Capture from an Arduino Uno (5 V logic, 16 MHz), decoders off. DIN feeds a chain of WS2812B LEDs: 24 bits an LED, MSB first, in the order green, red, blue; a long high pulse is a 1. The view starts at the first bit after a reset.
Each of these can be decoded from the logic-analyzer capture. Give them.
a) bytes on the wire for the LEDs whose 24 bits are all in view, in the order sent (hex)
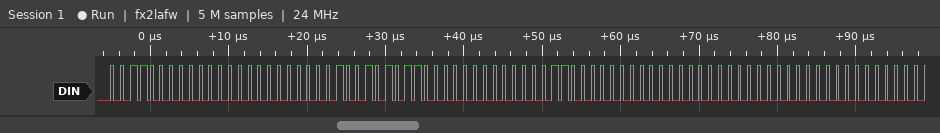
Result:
30 00 01 2B 00 06 00 00 00
